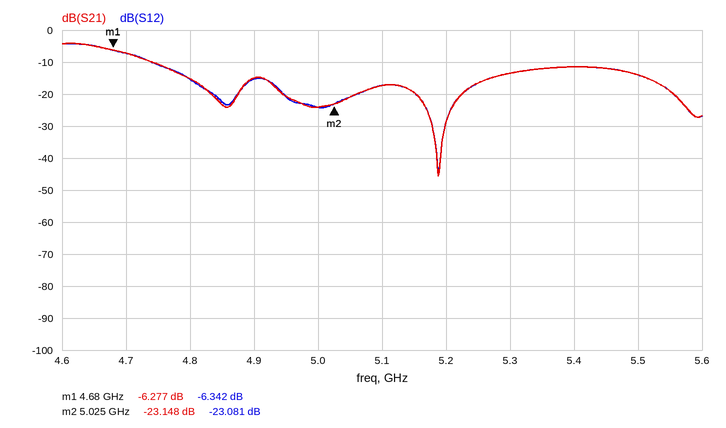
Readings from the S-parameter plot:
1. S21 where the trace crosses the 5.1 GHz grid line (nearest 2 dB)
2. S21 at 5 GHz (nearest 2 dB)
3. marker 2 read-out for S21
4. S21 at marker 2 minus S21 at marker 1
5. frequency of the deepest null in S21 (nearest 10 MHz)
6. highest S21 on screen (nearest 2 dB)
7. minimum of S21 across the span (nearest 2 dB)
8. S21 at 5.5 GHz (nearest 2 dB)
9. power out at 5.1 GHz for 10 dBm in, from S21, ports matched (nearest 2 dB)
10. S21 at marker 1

-18 dB
-24 dB
-23.148 dB
-16.871 dB
5.19 GHz
-4 dB
-46 dB
-14 dB
-8 dBm
-6.277 dB
